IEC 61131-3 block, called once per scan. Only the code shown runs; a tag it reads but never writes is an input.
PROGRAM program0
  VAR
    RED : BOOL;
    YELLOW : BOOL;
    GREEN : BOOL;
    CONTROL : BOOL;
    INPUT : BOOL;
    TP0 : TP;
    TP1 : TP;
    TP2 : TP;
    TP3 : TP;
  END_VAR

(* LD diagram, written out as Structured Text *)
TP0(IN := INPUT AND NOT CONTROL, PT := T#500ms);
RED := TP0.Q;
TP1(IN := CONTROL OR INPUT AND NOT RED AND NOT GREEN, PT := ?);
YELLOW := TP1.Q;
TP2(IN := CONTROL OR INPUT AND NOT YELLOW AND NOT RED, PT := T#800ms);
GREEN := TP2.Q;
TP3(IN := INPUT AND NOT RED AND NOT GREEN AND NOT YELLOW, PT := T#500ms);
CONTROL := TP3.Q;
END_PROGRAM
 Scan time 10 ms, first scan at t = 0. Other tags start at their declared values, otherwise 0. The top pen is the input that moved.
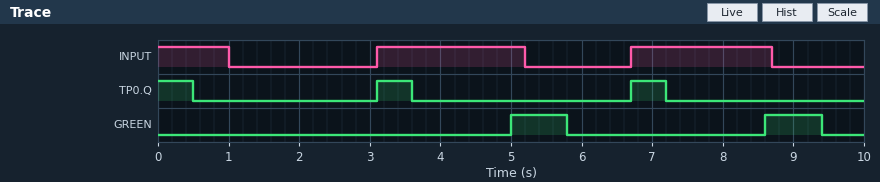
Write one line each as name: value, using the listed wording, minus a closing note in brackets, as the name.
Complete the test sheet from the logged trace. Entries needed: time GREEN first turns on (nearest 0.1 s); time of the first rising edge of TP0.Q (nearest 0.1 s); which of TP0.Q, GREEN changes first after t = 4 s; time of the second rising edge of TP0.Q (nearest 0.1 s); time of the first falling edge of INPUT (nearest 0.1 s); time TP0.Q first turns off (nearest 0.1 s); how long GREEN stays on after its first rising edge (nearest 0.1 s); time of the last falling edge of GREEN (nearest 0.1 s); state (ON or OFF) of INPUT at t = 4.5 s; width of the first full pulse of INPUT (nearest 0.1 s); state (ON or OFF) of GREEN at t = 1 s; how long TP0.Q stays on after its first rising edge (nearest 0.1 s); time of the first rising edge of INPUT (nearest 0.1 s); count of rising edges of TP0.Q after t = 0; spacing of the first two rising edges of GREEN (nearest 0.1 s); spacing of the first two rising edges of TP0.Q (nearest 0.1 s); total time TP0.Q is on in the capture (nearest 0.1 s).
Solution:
time GREEN first turns on: 5.0 s
time of the first rising edge of TP0.Q: 3.1 s
which of TP0.Q, GREEN changes first after t = 4 s: GREEN
time of the second rising edge of TP0.Q: 6.7 s
time of the first falling edge of INPUT: 1.0 s
time TP0.Q first turns off: 0.5 s
how long GREEN stays on after its first rising edge: 0.8 s
time of the last falling edge of GREEN: 9.4 s
state (ON or OFF) of INPUT at t = 4.5 s: ON
width of the first full pulse of INPUT: 2.1 s
state (ON or OFF) of GREEN at t = 1 s: OFF
how long TP0.Q stays on after its first rising edge: 0.5 s
time of the first rising edge of INPUT: 3.1 s
count of rising edges of TP0.Q after t = 0: 2
spacing of the first two rising edges of GREEN: 3.6 s
spacing of the first two rising edges of TP0.Q: 3.6 s
total time TP0.Q is on in the capture: 1.5 s
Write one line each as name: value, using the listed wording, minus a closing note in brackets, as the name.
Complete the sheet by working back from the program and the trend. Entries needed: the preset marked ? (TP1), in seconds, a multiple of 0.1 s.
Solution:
the preset marked ? (TP1), in seconds, a multiple of 0.1 s: 1.4 s
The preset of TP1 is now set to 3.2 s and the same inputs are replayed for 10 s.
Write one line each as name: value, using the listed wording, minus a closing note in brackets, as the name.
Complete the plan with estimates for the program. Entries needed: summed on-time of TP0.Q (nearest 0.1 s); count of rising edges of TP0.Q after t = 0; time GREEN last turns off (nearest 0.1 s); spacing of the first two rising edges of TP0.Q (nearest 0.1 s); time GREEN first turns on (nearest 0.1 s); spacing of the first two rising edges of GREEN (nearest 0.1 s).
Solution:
summed on-time of TP0.Q: 2.0 s
count of rising edges of TP0.Q after t = 0: 3
time GREEN last turns off: 8.5 s
spacing of the first two rising edges of TP0.Q: 1.9 s
time GREEN first turns on: 3.7 s
spacing of the first two rising edges of GREEN: 4.0 s
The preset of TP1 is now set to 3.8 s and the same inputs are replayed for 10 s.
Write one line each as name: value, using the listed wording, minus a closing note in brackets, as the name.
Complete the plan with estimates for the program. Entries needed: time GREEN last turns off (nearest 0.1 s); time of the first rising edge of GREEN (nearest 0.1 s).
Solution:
time GREEN last turns off: 5.1 s
time of the first rising edge of GREEN: 4.3 s
